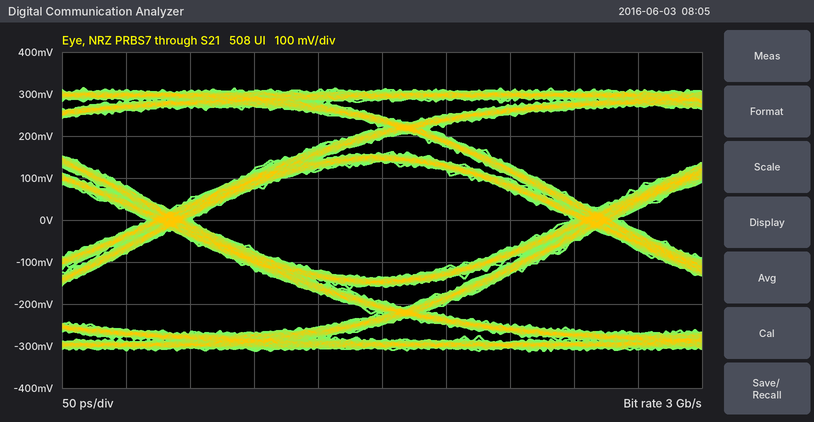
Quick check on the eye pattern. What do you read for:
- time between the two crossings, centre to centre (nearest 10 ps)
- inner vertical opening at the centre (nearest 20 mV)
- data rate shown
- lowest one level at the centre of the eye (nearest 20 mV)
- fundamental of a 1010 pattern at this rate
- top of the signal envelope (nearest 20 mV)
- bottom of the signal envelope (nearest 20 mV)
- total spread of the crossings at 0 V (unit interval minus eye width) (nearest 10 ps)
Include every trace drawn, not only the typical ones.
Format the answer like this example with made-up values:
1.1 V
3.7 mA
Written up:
330 ps
280 mV
3 Gb/s
140 mV
1.5 GHz
320 mV
-320 mV
40 ps
